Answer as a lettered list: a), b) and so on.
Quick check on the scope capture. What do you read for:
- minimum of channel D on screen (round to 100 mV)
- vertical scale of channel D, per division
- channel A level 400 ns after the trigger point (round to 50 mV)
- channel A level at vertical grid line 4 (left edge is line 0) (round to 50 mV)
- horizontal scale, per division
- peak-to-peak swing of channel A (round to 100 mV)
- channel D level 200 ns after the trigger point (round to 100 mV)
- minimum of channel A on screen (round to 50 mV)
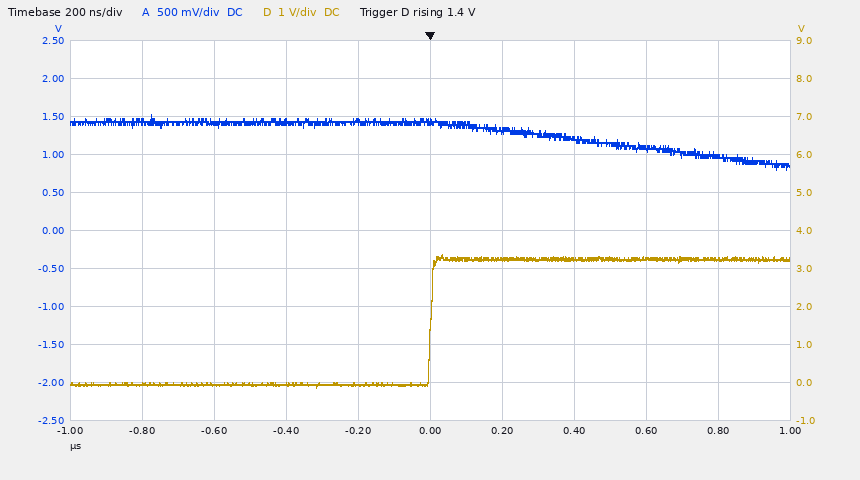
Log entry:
a) -100 mV
b) 1 V
c) 1.20 V
d) 1.45 V
e) 200 ns
f) 700 mV
g) 3.2 V
h) 800 mV
